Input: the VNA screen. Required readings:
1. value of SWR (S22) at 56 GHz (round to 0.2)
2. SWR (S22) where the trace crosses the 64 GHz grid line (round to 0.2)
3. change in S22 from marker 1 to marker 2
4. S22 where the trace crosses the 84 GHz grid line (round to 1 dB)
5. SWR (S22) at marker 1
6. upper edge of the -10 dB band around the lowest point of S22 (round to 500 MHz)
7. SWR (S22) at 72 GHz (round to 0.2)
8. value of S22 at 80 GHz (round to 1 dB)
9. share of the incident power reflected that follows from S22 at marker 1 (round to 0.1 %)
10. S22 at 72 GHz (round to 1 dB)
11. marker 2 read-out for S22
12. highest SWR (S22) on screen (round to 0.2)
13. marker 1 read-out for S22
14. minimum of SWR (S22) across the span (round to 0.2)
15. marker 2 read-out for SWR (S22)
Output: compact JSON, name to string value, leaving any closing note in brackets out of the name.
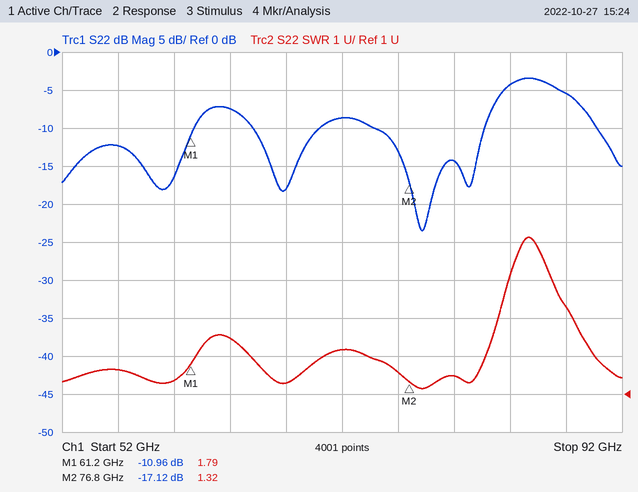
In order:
{"value of SWR (S22) at 56 GHz": "1.6", "SWR (S22) where the trace crosses the 64 GHz grid line": "2.4", "change in S22 from marker 1 to marker 2": "-6.16 dB", "S22 where the trace crosses the 84 GHz grid line": "-4 dB", "SWR (S22) at marker 1": "1.79", "upper edge of the -10 dB band around the lowest point of S22": "82.0 GHz", "SWR (S22) at 72 GHz": "2.2", "value of S22 at 80 GHz": "-14 dB", "share of the incident power reflected that follows from S22 at marker 1": "8.0 %", "S22 at 72 GHz": "-9 dB", "marker 2 read-out for S22": "-17.12 dB", "highest SWR (S22) on screen": "5.2", "marker 1 read-out for S22": "-10.96 dB", "minimum of SWR (S22) across the span": "1.2", "marker 2 read-out for SWR": "1.32"}
